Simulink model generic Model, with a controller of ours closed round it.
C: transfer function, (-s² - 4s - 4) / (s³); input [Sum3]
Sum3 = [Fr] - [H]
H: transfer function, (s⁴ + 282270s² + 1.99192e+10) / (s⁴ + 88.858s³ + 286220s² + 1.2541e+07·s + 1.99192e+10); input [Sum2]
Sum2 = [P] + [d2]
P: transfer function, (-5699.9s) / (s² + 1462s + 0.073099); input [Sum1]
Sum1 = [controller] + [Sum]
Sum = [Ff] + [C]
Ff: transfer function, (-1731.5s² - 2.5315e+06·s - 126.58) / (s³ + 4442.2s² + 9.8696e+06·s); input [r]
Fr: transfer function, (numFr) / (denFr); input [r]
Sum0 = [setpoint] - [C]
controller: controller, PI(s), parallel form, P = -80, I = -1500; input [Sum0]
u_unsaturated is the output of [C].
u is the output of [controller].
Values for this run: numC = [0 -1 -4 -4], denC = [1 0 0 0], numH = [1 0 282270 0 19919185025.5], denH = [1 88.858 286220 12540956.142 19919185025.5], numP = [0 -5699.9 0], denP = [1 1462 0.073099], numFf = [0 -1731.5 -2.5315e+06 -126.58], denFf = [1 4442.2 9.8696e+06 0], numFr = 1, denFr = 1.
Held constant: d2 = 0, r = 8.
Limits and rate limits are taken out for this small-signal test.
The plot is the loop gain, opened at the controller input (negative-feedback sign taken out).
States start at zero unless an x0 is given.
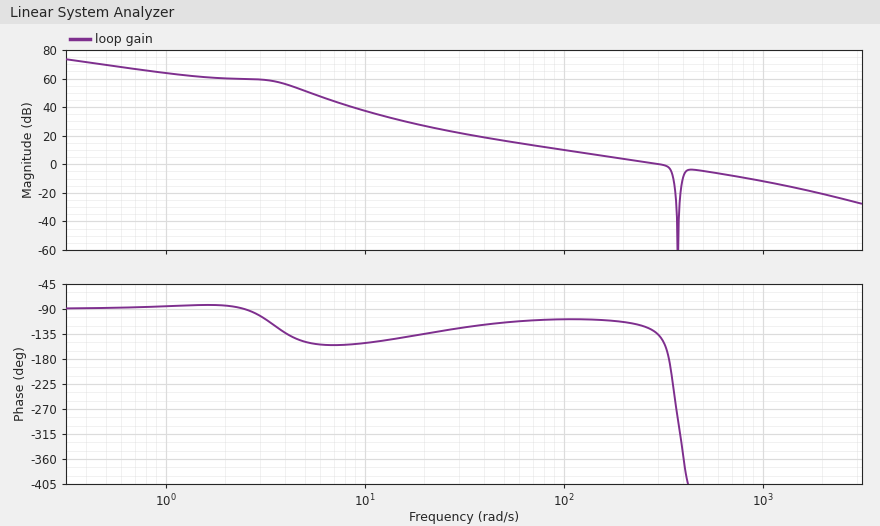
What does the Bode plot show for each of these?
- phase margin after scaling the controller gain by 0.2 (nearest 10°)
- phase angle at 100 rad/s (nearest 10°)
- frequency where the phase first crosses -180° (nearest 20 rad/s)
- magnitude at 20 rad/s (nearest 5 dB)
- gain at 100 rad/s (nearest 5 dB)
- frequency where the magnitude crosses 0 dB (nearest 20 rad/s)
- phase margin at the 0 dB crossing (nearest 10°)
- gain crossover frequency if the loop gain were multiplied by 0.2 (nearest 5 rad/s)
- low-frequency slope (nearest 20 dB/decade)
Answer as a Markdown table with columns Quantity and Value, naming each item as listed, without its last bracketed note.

| Quantity | Value |
|---|---|
| phase margin after scaling the controller gain by 0.2 | 70° |
| phase angle at 100 rad/s | -110° |
| frequency where the phase first crosses -180° | 340 rad/s |
| magnitude at 20 rad/s | 25 dB |
| gain at 100 rad/s | 10 dB |
| frequency where the magnitude crosses 0 dB | 300 rad/s |
| phase margin at the 0 dB crossing | 40° |
| gain crossover frequency if the loop gain were multiplied by 0.2 | 65 rad/s |
| low-frequency slope | -20 dB/decade |
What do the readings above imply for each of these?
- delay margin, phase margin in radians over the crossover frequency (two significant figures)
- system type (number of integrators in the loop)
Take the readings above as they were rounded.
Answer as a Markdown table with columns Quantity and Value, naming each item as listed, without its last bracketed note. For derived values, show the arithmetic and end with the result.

| Quantity | Value |
|---|---|
| delay margin, phase margin in radians over the crossover frequency | 40 × π / 180 / 300 = 0.0023 s |
| system type | 1 |
